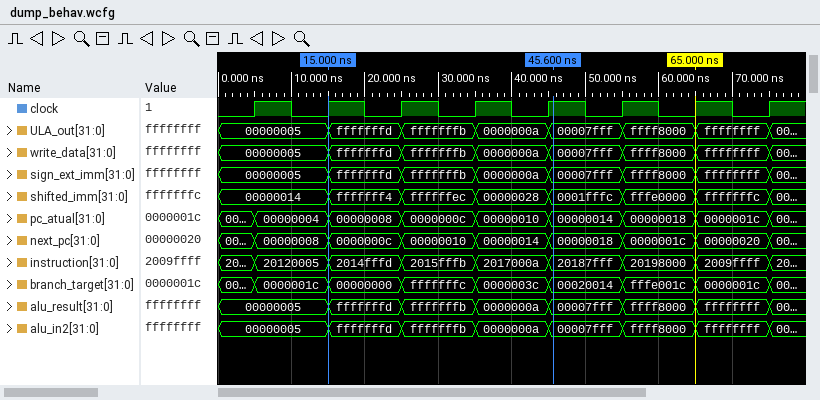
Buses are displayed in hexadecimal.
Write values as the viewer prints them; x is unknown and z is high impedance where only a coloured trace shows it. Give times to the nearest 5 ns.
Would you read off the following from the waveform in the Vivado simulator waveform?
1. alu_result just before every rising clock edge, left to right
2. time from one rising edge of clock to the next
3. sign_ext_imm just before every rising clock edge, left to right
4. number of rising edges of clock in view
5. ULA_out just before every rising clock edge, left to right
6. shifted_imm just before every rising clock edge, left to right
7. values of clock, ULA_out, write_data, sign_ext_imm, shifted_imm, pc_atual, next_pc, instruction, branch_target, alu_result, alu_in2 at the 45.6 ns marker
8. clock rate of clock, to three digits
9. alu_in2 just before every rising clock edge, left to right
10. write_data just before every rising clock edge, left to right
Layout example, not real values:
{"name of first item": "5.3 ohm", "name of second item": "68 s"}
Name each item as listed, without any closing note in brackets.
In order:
{"alu_result just before every rising clock edge, left to right": "00000005, 00000005, fffffffd, fffffffb, 0000000a, 00007fff, ffff8000, ffffffff", "time from one rising edge of clock to the next": "10 ns", "sign_ext_imm just before every rising clock edge, left to right": "00000005, 00000005, fffffffd, fffffffb, 0000000a, 00007fff, ffff8000, ffffffff", "number of rising edges of clock in view": "8", "ULA_out just before every rising clock edge, left to right": "00000005, 00000005, fffffffd, fffffffb, 0000000a, 00007fff, ffff8000, ffffffff", "shifted_imm just before every rising clock edge, left to right": "00000014, 00000014, fffffff4, ffffffec, 00000028, 0001fffc, fffe0000, fffffffc", "values of clock, ULA_out, write_data, sign_ext_imm, shifted_imm, pc_atual, next_pc, instruction, branch_target, alu_result, alu_in2 at the 45.6 ns marker": "clock=1, ULA_out=00007fff, write_data=00007fff, sign_ext_imm=00007fff, shifted_imm=0001fffc, pc_atual=00000014, next_pc=00000018, instruction=20187fff, branch_target=00020014, alu_result=00007fff, alu_in2=00007fff", "clock rate of clock, to three digits": "100 MHz", "alu_in2 just before every rising clock edge, left to right": "00000005, 00000005, fffffffd, fffffffb, 0000000a, 00007fff, ffff8000, ffffffff", "write_data just before every rising clock edge, left to right": "00000005, 00000005, fffffffd, fffffffb, 0000000a, 00007fff, ffff8000, ffffffff"}
